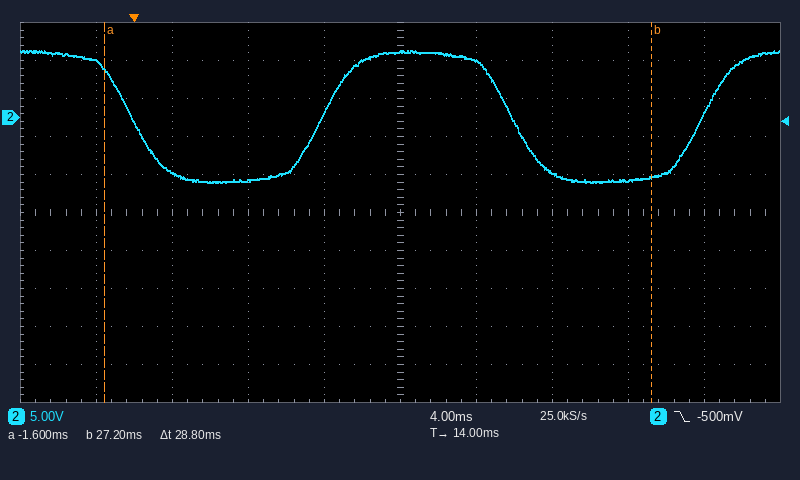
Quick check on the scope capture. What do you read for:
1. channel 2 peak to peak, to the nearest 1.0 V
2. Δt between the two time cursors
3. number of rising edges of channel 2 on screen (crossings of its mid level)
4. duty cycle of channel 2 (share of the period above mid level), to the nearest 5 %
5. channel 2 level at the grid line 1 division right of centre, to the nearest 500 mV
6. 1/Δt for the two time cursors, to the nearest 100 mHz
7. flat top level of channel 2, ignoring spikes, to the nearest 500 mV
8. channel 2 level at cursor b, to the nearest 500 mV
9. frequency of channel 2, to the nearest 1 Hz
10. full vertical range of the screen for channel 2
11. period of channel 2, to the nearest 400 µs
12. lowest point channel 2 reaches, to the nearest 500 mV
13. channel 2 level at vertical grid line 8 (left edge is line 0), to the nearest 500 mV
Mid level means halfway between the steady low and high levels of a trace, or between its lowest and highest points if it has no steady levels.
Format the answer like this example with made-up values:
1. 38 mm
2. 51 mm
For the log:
1. 17.0 V
2. 28.8 ms
3. 2
4. 50 %
5. 7.5 V
6. 34.7 Hz
7. 8.5 V
8. -8.0 V
9. 50 Hz
10. 50 V
11. 20.0 ms
12. -8.5 V
13. -8.5 V
